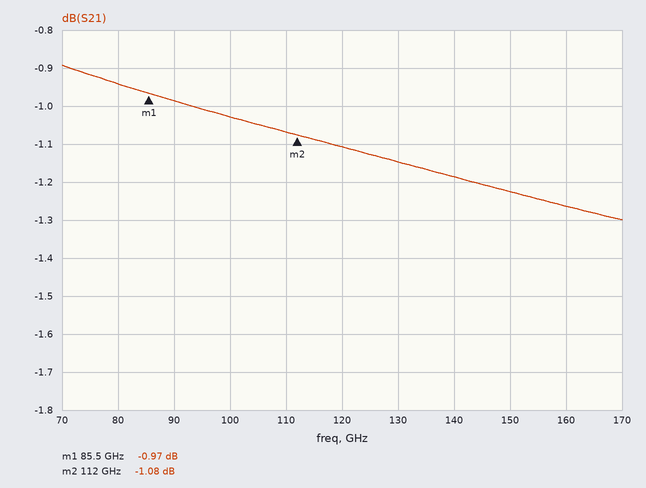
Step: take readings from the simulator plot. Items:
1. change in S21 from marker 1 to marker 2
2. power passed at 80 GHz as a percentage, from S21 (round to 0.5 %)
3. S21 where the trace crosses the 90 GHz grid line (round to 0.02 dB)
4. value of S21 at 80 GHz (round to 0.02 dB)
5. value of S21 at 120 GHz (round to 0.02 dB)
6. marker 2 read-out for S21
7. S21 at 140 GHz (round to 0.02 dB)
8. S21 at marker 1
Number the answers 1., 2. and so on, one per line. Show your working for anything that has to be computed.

1. -1.08 − (-0.97) = -0.11 dB
2. 10^(-0.94/10) ≈ 80.5 %
3. -0.98 dB
4. -0.94 dB
5. -1.10 dB
6. -1.08 dB
7. -1.18 dB
8. -0.97 dB
